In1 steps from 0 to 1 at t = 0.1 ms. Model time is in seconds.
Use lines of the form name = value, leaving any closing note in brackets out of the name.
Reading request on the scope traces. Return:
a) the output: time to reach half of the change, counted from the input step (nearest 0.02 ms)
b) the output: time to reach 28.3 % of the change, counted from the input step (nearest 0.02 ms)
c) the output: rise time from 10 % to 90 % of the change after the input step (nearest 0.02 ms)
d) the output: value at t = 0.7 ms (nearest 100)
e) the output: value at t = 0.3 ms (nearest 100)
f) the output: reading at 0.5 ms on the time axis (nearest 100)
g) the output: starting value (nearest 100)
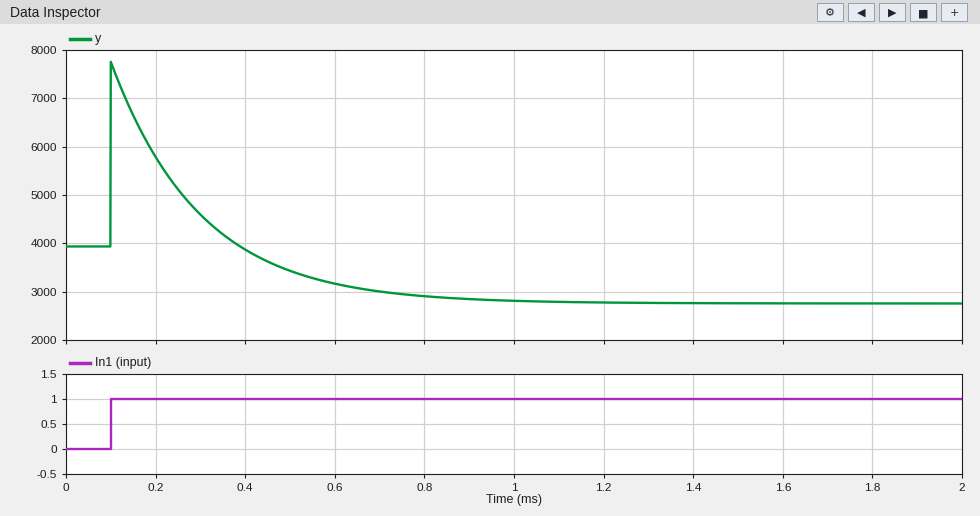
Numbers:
the output: time to reach half of the change, counted from the input step = 0.42 ms
the output: time to reach 28.3 % of the change, counted from the input step = 0.36 ms
the output: rise time from 10 % to 90 % of the change after the input step = 0.44 ms
the output: value at t = 0.7 ms = 3000
the output: value at t = 0.3 ms = 4600
the output: reading at 0.5 ms on the time axis = 3400
the output: starting value = 3900
